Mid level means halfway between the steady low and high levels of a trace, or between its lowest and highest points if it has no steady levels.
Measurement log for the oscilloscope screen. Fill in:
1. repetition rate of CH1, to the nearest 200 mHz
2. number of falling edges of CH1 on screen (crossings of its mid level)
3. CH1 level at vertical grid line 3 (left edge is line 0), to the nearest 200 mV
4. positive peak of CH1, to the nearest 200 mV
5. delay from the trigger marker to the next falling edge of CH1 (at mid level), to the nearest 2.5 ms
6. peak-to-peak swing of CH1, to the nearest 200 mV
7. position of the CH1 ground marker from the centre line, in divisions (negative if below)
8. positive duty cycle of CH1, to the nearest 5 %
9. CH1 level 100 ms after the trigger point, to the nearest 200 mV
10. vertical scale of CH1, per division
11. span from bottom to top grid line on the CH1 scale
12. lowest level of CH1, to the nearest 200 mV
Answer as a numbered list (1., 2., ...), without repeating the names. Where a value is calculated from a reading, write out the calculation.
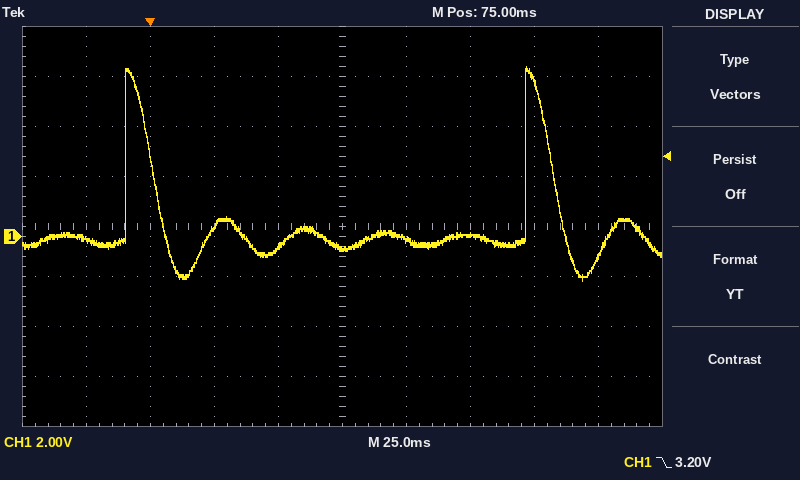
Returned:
1. 6.4 Hz
2. 2
3. 400 mV
4. 6.8 V
5. 157.5 ms
6. 6.8 V − (-1.8 V) = 8.6 V
7. -0.2 div
8. 5 %
9. -200 mV
10. 2 V
11. 16 V
12. -1.8 V
